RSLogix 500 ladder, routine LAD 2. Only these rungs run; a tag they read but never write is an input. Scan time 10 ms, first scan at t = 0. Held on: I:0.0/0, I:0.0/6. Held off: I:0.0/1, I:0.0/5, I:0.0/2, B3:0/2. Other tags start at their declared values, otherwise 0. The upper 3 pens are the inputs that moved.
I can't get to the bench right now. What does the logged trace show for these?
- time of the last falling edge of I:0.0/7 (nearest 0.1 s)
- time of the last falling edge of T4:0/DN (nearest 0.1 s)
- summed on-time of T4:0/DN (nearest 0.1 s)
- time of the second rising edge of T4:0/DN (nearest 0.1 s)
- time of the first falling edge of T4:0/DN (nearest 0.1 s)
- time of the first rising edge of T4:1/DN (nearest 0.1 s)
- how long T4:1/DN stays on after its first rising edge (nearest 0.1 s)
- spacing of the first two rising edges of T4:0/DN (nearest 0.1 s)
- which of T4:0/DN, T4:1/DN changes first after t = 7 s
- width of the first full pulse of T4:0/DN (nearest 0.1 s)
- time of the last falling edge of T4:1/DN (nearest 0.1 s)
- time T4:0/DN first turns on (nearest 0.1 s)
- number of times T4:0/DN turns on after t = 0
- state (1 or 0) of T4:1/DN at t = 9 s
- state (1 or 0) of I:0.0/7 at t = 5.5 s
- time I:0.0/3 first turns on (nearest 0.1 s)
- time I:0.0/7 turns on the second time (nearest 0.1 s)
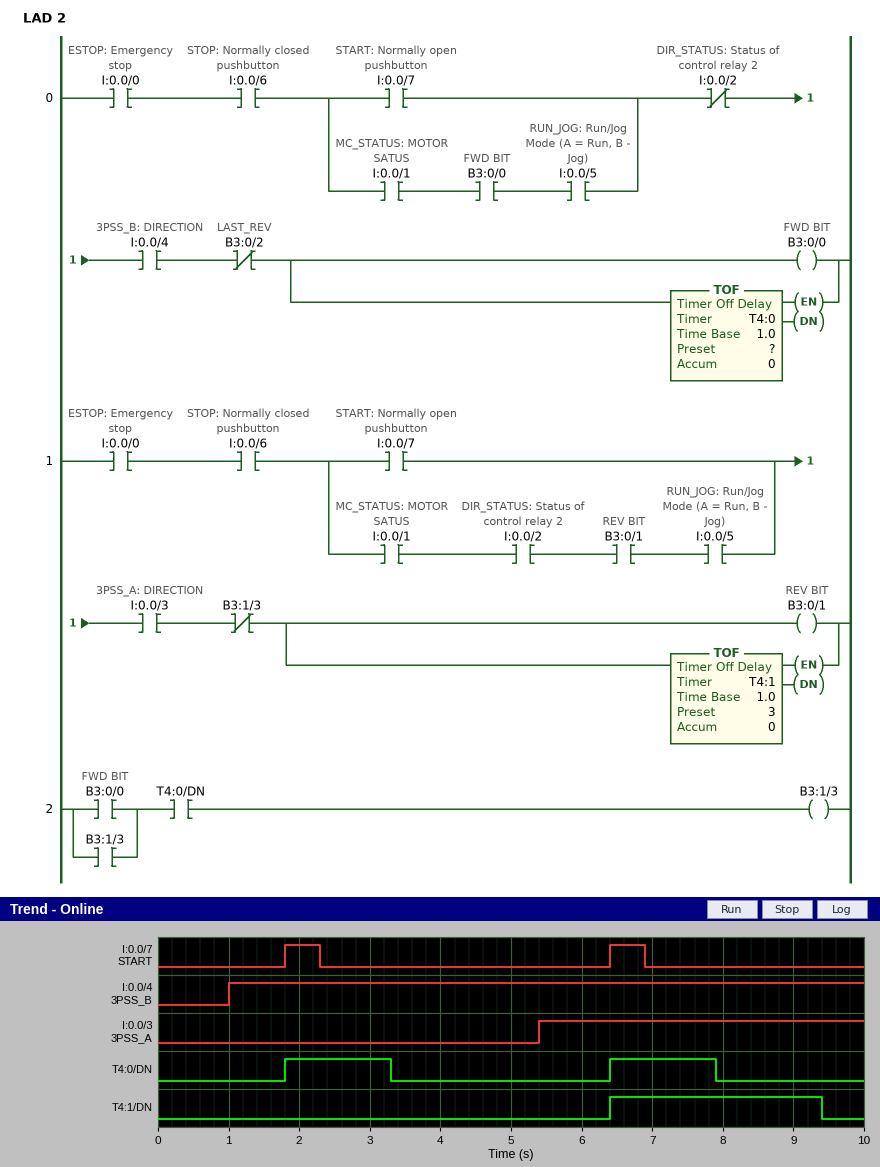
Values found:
6.9 s
7.9 s
3.0 s
6.4 s
3.3 s
6.4 s
3.0 s
4.6 s
T4:0/DN
1.5 s
9.4 s
1.8 s
2
1
0
5.4 s
6.4 s
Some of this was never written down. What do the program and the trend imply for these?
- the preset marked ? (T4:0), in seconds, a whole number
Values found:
1 s
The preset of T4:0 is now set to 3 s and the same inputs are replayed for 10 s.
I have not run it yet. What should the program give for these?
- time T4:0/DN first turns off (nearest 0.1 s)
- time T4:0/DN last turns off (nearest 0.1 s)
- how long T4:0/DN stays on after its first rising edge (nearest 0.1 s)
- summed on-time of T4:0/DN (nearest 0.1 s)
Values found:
5.3 s
9.9 s
3.5 s
7.0 s
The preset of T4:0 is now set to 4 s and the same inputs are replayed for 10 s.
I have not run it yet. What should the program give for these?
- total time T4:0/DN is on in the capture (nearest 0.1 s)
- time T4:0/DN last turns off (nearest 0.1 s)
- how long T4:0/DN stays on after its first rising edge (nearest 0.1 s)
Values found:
8.1 s
6.3 s
4.5 s
